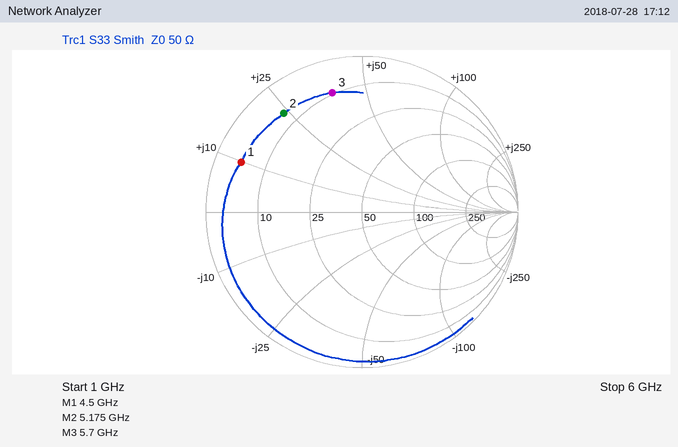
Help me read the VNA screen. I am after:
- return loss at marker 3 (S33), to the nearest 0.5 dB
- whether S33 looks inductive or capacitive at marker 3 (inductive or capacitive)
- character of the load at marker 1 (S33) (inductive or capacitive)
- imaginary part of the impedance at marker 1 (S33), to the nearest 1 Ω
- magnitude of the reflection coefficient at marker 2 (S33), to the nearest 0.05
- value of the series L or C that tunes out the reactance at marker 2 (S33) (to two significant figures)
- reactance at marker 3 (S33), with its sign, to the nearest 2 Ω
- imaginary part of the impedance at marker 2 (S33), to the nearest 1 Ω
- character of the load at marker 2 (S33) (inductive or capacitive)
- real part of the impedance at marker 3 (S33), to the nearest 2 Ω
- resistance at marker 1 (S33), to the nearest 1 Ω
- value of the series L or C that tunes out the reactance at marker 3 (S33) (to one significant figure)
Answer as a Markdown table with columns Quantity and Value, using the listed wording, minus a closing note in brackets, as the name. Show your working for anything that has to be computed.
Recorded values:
| Quantity | Value |
|---|---|
| return loss at marker 3 (S33), to the nearest 0.5 dB | 2.0 dB |
| whether S33 looks inductive or capacitive at marker 3 | inductive |
| character of the load at marker 1 (S33) | inductive |
| imaginary part of the impedance at marker 1 (S33), to the nearest 1 Ω | +10 Ω |
| magnitude of the reflection coefficient at marker 2 (S33), to the nearest 0.05 | 0.80 |
| value of the series L or C that tunes out the reactance at marker 2 (S33) | C = 1/(2π × 5.175 GHz × 24 Ω) ≈ 1.3 pF |
| reactance at marker 3 (S33), with its sign, to the nearest 2 Ω | +38 Ω |
| imaginary part of the impedance at marker 2 (S33), to the nearest 1 Ω | +24 Ω |
| character of the load at marker 2 (S33) | inductive |
| real part of the impedance at marker 3 (S33), to the nearest 2 Ω | 10 Ω |
| resistance at marker 1 (S33), to the nearest 1 Ω | 5 Ω |
| value of the series L or C that tunes out the reactance at marker 3 (S33) | C = 1/(2π × 5.7 GHz × 38 Ω) ≈ 735 fF, so 700 fF to one significant figure |
